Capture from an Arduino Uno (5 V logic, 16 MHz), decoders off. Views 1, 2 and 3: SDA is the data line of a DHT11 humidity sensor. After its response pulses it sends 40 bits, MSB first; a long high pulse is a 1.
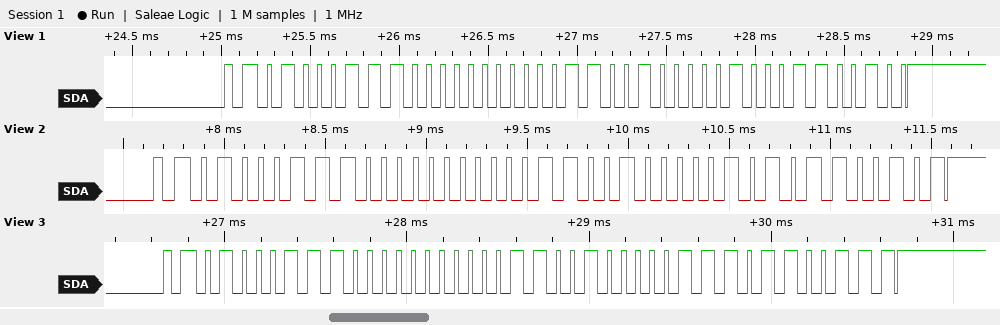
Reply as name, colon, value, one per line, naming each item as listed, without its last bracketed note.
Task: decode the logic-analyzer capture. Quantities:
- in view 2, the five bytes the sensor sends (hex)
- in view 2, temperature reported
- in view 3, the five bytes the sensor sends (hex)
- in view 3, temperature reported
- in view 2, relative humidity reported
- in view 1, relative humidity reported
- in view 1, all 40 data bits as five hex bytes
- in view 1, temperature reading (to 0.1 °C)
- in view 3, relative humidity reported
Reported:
in view 2, the five bytes the sensor sends: 47 00 19 05 65
in view 2, temperature reported: 25.5 °C
in view 3, the five bytes the sensor sends: 47 00 19 07 67
in view 3, temperature reported: 25.7 °C
in view 2, relative humidity reported: 71 %
in view 1, relative humidity reported: 71 %
in view 1, all 40 data bits as five hex bytes: 47 00 19 04 64
in view 1, temperature reading: 25.4 °C
in view 3, relative humidity reported: 71 %
